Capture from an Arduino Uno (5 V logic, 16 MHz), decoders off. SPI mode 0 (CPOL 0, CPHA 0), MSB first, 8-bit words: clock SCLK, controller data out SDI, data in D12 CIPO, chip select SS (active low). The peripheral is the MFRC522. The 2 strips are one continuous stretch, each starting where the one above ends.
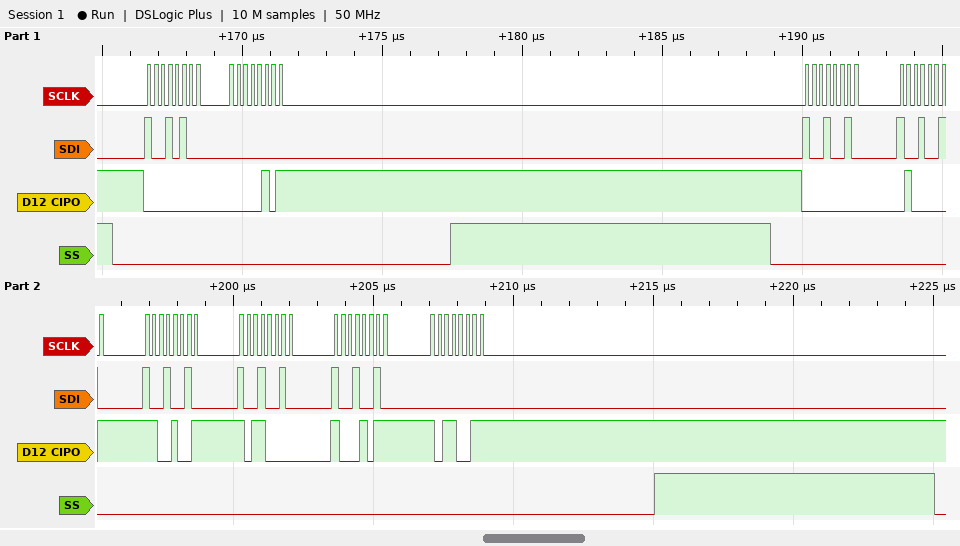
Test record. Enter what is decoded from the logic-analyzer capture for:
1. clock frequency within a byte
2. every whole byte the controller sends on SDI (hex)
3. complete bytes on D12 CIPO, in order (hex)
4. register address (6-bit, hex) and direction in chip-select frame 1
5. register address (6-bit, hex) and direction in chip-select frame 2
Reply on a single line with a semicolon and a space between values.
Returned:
4 MHz; 94 00 92 92 92 92 92 00; 00 05 00 41 C9 B0 8B B3; 0x0A read; 0x09 read
